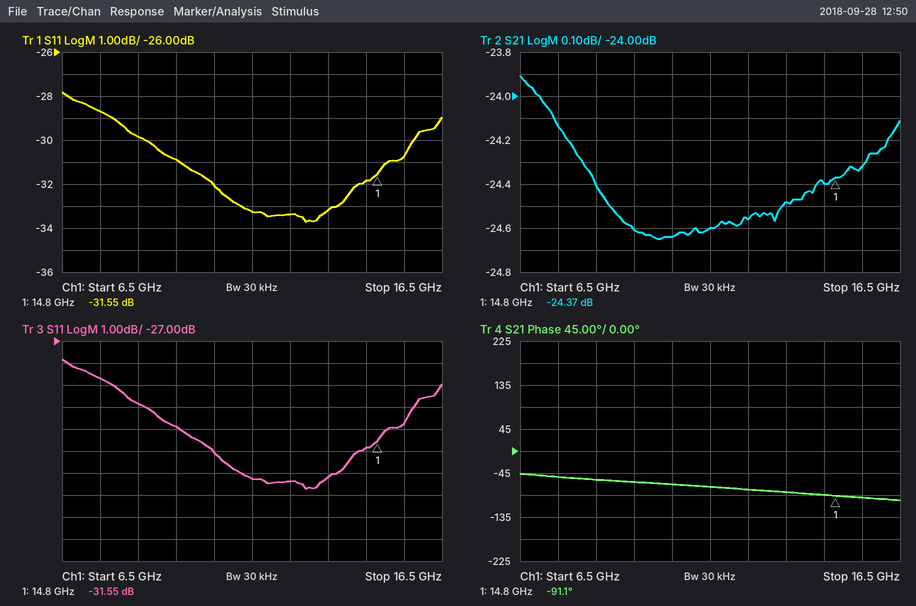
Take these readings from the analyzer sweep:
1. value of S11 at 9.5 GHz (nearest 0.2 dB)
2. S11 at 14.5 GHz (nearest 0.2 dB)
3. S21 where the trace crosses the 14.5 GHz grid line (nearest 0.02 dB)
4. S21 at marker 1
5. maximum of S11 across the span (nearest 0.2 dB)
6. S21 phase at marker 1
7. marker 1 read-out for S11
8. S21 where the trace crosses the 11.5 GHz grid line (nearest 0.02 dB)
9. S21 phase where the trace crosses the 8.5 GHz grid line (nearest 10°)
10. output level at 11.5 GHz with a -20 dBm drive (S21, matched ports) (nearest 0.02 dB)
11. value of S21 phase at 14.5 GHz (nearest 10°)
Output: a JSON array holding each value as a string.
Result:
["-30.8 dB", "-31.8 dB", "-24.40 dB", "-24.37 dB", "-27.8 dB", "-91.1°", "-31.55 dB", "-24.60 dB", "-60°", "-44.60 dBm", "-90°"]
